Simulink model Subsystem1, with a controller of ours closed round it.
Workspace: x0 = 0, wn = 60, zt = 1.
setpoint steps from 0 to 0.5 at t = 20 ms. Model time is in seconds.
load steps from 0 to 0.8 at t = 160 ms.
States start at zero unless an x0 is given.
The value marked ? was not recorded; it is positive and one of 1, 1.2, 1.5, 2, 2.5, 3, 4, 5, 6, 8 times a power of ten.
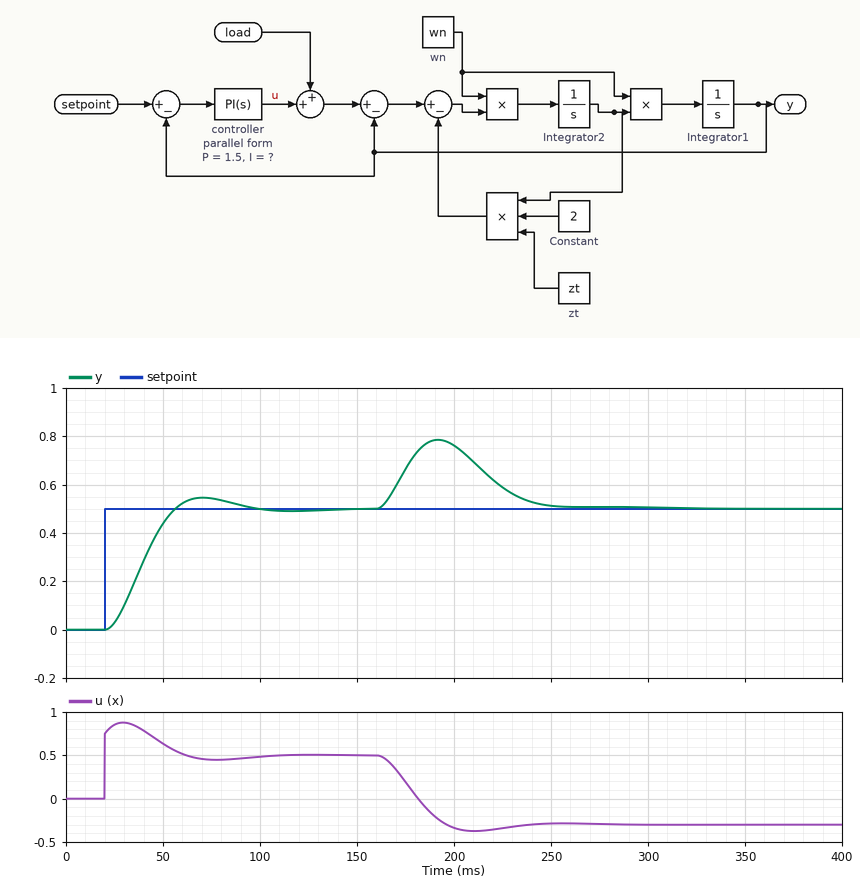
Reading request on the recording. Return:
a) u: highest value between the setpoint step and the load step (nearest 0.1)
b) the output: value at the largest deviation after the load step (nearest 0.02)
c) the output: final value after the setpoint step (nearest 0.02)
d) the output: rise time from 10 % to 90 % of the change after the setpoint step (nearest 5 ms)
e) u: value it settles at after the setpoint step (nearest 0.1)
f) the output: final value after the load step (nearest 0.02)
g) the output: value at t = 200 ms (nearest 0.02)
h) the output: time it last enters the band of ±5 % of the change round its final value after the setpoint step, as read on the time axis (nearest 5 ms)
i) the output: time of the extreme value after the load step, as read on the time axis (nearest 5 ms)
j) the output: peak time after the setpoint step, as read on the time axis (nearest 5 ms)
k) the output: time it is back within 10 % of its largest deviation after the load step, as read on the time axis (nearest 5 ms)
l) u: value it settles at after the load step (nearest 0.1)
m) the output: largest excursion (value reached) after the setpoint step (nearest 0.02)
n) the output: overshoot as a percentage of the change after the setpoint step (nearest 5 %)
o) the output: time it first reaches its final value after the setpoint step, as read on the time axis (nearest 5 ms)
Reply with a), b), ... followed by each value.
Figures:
a) 0.9
b) 0.78
c) 0.50
d) 25 ms
e) 0.5
f) 0.50
g) 0.76
h) 85 ms
i) 190 ms
j) 70 ms
k) 240 ms
l) -0.3
m) 0.54
n) 10 %
o) 55 ms
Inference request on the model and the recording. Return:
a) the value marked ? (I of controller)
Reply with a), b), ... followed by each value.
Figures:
a) 60
